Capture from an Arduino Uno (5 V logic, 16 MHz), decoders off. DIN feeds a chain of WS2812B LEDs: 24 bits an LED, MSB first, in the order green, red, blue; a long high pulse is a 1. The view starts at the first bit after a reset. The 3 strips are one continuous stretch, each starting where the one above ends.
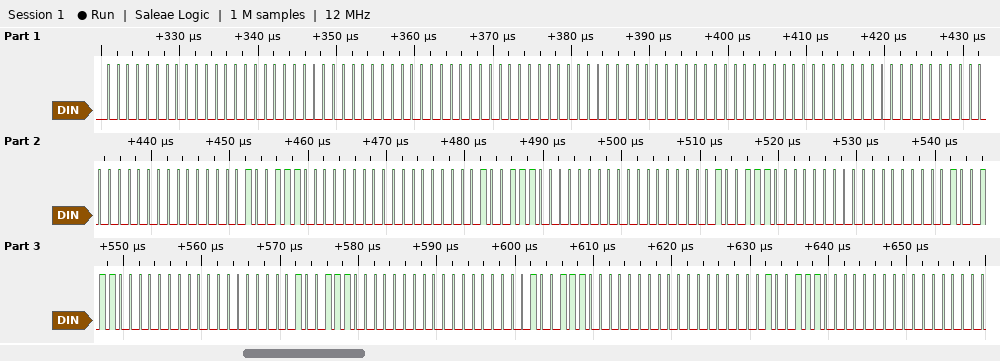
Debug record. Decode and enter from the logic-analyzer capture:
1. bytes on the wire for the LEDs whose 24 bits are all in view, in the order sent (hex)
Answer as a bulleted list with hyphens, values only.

- 00 00 00 00 00 00 00 00 00 00 00 00 00 4E 00 00 4E 00 00 4E 00 00 4E 00 00 4E 00 00 4E 00 00 4E 00
